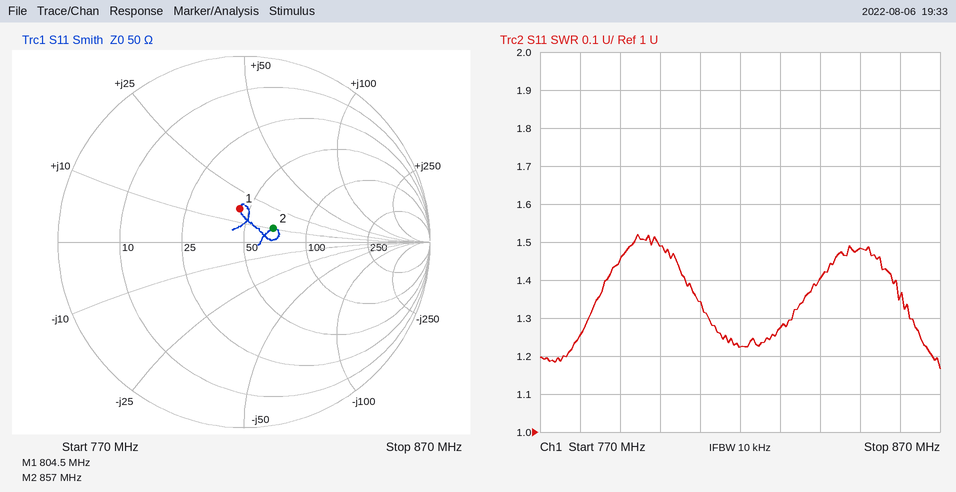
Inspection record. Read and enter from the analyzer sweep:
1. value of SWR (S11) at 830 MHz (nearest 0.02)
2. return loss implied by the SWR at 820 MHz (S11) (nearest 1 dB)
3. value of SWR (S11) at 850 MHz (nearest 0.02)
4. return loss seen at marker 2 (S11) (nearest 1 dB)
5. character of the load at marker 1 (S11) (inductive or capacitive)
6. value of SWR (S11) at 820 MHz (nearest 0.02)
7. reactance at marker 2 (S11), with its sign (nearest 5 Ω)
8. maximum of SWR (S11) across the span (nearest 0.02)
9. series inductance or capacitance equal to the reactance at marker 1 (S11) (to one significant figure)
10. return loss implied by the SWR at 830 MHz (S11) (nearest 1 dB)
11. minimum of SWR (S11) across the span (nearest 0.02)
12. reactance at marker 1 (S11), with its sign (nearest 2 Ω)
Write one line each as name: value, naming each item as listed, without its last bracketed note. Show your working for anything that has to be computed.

value of SWR (S11) at 830 MHz: 1.28
return loss implied by the SWR at 820 MHz (S11): −20 log10((1.22 − 1)/(1.22 + 1)) ≈ 20 dB
value of SWR (S11) at 850 MHz: 1.48
return loss seen at marker 2 (S11): 15 dB
character of the load at marker 1 (S11): inductive
value of SWR (S11) at 820 MHz: 1.22
reactance at marker 2 (S11), with its sign: +10 Ω
maximum of SWR (S11) across the span: 1.52
series inductance or capacitance equal to the reactance at marker 1 (S11): L = 16 Ω/(2π × 804.5 MHz) ≈ 3 nH
return loss implied by the SWR at 830 MHz (S11): −20 log10((1.28 − 1)/(1.28 + 1)) ≈ 18 dB
minimum of SWR (S11) across the span: 1.16
reactance at marker 1 (S11), with its sign: +16 Ω
